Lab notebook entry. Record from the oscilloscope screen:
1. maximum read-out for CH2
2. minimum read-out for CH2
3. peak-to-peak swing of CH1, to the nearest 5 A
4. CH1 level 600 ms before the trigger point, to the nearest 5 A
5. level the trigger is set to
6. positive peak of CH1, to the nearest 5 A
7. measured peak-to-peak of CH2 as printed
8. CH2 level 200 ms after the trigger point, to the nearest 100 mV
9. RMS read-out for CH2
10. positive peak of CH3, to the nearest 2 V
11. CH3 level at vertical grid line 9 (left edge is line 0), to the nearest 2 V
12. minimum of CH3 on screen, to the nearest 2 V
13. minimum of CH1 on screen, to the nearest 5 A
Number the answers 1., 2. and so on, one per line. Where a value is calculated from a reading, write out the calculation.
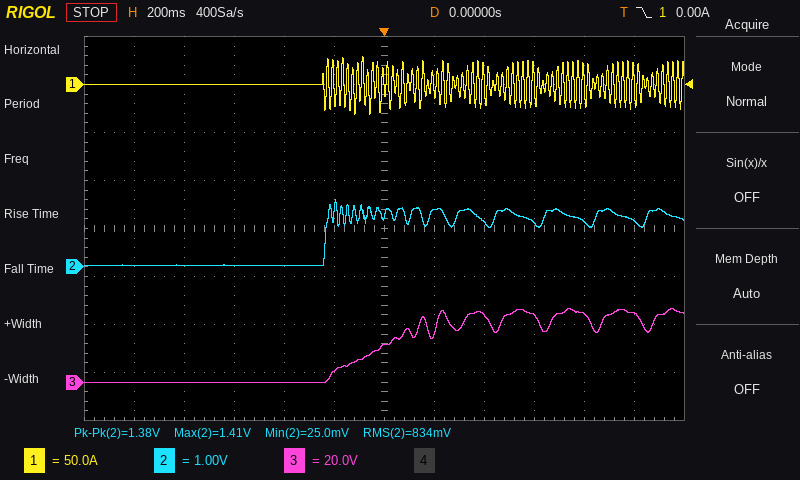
1. 1.41 V
2. 25.0 mV
3. 30 A − (-30 A) = 60 A
4. 0 A
5. 0.00 A
6. 30 A
7. 1.38 V
8. 1.2 V
9. 834 mV
10. 30 V
11. 28 V
12. 0 V
13. -30 A
